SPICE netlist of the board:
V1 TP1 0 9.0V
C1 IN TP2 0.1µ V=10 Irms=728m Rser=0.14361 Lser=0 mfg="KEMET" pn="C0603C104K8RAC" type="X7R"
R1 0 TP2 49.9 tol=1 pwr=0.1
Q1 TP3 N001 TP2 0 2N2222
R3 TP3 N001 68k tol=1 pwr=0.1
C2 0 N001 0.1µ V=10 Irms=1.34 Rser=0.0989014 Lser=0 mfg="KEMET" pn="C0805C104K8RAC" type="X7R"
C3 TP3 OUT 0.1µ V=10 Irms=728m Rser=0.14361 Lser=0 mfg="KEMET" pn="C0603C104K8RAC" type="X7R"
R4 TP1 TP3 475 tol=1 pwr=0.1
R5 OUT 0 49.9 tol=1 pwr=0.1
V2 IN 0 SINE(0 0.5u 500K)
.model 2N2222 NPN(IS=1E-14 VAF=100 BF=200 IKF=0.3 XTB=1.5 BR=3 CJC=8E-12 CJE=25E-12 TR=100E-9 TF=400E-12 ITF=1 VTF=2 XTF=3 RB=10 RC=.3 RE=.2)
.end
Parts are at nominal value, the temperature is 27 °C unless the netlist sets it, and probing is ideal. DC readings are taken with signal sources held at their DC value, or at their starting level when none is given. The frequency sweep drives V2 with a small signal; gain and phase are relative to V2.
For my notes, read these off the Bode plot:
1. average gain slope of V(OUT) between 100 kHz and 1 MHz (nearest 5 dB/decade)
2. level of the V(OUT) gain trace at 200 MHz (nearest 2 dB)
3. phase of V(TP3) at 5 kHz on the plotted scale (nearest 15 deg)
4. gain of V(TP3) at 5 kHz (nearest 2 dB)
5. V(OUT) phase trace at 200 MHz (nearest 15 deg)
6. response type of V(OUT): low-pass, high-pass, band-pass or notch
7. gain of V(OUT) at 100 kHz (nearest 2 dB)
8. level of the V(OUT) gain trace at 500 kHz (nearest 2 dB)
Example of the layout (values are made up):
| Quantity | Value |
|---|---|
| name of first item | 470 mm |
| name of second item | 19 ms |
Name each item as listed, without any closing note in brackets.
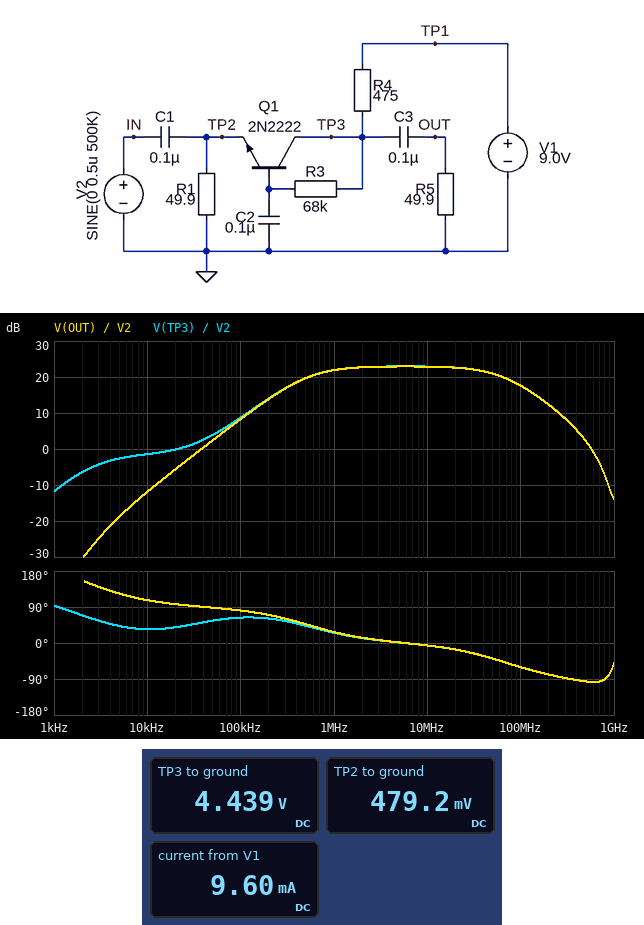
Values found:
| Quantity | Value |
|---|---|
| average gain slope of V(OUT) between 100 kHz and 1 MHz | 15 dB/decade |
| level of the V(OUT) gain trace at 200 MHz | 12 dB |
| phase of V(TP3) at 5 kHz on the plotted scale | 45 deg |
| gain of V(TP3) at 5 kHz | -2 dB |
| V(OUT) phase trace at 200 MHz | -75 deg |
| response type of V(OUT): low-pass, high-pass, band-pass or notch | band-pass |
| gain of V(OUT) at 100 kHz | 8 dB |
| level of the V(OUT) gain trace at 500 kHz | 20 dB |
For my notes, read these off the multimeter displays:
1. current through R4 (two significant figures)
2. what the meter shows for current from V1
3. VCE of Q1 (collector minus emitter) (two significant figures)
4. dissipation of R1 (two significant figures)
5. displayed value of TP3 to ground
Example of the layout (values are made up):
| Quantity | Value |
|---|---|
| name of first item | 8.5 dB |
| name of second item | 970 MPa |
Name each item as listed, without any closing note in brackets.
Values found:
| Quantity | Value |
|---|---|
| current through R4 | 9.6 mA |
| what the meter shows for current from V1 | 9.60 mA |
| VCE of Q1 (collector minus emitter) | 4.0 V |
| dissipation of R1 | 4.6 mW |
| displayed value of TP3 to ground | 4.439 V |
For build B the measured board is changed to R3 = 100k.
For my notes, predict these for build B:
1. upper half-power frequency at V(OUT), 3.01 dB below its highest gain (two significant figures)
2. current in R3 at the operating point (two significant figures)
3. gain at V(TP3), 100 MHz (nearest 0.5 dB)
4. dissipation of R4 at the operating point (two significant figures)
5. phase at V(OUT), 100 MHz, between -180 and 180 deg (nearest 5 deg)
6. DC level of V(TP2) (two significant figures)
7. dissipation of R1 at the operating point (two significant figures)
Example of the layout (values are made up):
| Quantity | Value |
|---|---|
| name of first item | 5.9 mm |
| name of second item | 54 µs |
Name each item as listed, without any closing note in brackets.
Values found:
| Quantity | Value |
|---|---|
| upper half-power frequency at V(OUT), 3.01 dB below its highest gain | 73 MHz |
| current in R3 at the operating point | 40 µA |
| gain at V(TP3), 100 MHz | 17.0 dB |
| dissipation of R4 at the operating point | 32 mW |
| phase at V(OUT), 100 MHz, between -180 and 180 deg | -55 deg |
| DC level of V(TP2) | 410 mV |
| dissipation of R1 at the operating point | 3.3 mW |
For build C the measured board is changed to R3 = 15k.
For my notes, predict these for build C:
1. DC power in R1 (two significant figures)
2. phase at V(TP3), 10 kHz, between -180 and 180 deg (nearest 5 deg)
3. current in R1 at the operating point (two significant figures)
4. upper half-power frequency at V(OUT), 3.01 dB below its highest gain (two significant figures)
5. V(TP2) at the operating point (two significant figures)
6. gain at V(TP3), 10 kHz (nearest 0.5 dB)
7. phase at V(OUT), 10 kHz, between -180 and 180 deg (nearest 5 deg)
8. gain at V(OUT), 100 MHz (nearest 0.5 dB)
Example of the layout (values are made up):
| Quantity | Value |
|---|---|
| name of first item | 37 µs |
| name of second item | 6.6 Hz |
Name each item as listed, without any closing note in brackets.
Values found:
| Quantity | Value |
|---|---|
| DC power in R1 | 9.4 mW |
| phase at V(TP3), 10 kHz, between -180 and 180 deg | 35 deg |
| current in R1 at the operating point | 14 mA |
| upper half-power frequency at V(OUT), 3.01 dB below its highest gain | 47 MHz |
| V(TP2) at the operating point | 690 mV |
| gain at V(TP3), 10 kHz | -1.0 dB |
| phase at V(OUT), 10 kHz, between -180 and 180 deg | 110 deg |
| gain at V(OUT), 100 MHz | 18.0 dB |
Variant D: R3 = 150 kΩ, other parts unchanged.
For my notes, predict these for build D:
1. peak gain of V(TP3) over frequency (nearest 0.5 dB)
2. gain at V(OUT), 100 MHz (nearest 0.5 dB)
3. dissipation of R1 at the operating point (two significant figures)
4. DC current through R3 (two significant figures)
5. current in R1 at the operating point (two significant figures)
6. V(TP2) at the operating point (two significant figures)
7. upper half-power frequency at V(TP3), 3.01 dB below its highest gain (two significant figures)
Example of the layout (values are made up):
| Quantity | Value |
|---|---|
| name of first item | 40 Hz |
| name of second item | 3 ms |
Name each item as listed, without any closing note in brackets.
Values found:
| Quantity | Value |
|---|---|
| peak gain of V(TP3) over frequency | 20.0 dB |
| gain at V(OUT), 100 MHz | 16.5 dB |
| dissipation of R1 at the operating point | 2.2 mW |
| DC current through R3 | 32 µA |
| current in R1 at the operating point | 6.6 mA |
| V(TP2) at the operating point | 330 mV |
| upper half-power frequency at V(TP3), 3.01 dB below its highest gain | 85 MHz |
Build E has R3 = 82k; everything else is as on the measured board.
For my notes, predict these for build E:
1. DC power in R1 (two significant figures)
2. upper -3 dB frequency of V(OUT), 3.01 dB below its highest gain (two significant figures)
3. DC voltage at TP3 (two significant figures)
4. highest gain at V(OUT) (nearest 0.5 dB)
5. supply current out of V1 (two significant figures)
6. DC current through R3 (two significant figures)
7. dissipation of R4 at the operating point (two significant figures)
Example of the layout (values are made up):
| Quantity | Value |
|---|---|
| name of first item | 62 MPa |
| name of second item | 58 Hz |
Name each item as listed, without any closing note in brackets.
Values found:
| Quantity | Value |
|---|---|
| DC power in R1 | 4.0 mW |
| upper -3 dB frequency of V(OUT), 3.01 dB below its highest gain | 69 MHz |
| DC voltage at TP3 | 4.8 V |
| highest gain at V(OUT) | 22.5 dB |
| supply current out of V1 | 8.9 mA |
| DC current through R3 | 44 µA |
| dissipation of R4 at the operating point | 38 mW |
